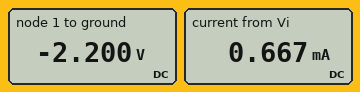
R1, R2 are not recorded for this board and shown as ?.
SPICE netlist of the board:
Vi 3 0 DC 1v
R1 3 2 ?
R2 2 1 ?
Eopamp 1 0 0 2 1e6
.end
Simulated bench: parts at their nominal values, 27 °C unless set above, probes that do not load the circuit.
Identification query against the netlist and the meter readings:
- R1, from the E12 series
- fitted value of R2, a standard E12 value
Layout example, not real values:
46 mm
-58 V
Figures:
1.5 kΩ
3.3 kΩ
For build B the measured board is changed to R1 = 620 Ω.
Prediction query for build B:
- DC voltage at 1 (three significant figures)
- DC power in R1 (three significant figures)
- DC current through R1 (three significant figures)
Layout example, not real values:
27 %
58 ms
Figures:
-5.32 V
1.61 mW
1.61 mA
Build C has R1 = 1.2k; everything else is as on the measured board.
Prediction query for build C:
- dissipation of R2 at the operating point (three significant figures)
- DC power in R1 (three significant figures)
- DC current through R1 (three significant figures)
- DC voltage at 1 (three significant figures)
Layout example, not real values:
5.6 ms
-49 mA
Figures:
2.29 mW
833 µW
833 µA
-2.75 V
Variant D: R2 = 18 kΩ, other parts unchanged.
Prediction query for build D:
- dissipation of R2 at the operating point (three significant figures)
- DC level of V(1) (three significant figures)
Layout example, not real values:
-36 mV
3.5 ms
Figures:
8.00 mW
-12.0 V
